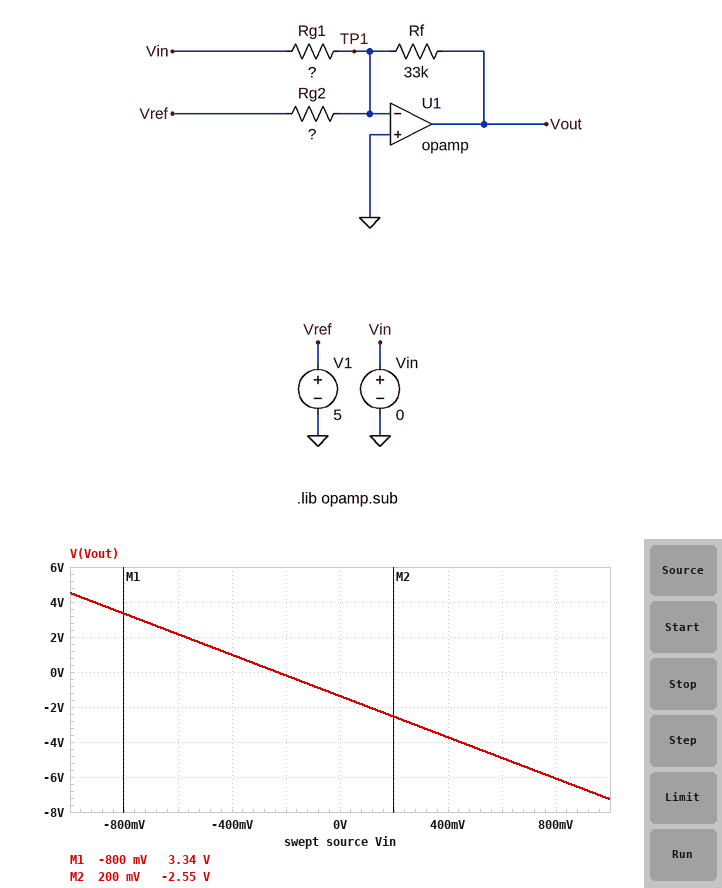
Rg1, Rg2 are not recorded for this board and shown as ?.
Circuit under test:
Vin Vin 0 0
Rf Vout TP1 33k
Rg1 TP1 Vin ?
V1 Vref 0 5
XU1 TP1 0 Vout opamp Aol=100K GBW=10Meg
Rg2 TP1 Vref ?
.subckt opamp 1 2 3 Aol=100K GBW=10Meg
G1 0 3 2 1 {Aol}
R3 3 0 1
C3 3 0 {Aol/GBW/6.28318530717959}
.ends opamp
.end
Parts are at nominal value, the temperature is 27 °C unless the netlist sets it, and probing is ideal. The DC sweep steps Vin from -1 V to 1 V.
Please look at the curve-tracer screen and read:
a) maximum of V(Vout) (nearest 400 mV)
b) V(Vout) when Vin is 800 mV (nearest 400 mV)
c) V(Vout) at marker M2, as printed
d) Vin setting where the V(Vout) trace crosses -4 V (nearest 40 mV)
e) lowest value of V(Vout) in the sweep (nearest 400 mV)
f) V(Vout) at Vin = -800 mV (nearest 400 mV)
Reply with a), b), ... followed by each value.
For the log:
a) 4.4 V
b) -6.0 V
c) -2.55 V
d) 440 mV
e) -7.2 V
f) 3.2 V
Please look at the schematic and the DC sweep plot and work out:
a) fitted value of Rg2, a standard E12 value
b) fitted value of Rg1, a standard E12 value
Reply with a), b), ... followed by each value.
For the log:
a) 120 kΩ
b) 5.6 kΩ
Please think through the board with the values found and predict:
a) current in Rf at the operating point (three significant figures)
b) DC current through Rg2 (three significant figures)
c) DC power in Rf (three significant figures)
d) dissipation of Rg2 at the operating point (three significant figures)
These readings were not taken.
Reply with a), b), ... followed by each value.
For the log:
a) 41.7 µA
b) 41.7 µA
c) 57.3 µW
d) 208 µW
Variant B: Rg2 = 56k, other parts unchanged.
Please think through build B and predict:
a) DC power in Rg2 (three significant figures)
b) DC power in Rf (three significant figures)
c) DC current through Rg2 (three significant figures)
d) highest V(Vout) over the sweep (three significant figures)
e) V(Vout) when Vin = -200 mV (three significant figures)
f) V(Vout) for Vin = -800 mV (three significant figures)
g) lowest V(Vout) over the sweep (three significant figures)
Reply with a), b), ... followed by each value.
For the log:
a) 446 µW
b) 263 µW
c) 89.3 µA
d) 2.95 V
e) -1.77 V
f) 1.77 V
g) -8.84 V
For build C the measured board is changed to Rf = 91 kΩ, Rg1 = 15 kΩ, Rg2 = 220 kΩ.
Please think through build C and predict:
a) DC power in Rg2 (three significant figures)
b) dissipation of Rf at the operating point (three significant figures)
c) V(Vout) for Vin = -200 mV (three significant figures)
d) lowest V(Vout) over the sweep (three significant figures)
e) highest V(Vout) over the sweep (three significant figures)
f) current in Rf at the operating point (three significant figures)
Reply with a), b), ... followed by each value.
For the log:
a) 114 µW
b) 47.0 µW
c) -855 mV
d) -8.13 V
e) 4.00 V
f) 22.7 µA
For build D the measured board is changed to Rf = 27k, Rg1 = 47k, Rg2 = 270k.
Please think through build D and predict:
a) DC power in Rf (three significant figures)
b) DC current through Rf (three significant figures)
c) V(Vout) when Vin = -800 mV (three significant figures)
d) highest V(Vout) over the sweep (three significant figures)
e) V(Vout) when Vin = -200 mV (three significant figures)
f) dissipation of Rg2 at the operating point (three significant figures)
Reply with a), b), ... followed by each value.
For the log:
a) 9.26 µW
b) 18.5 µA
c) -40.4 mV
d) 74.5 mV
e) -385 mV
f) 92.6 µW
